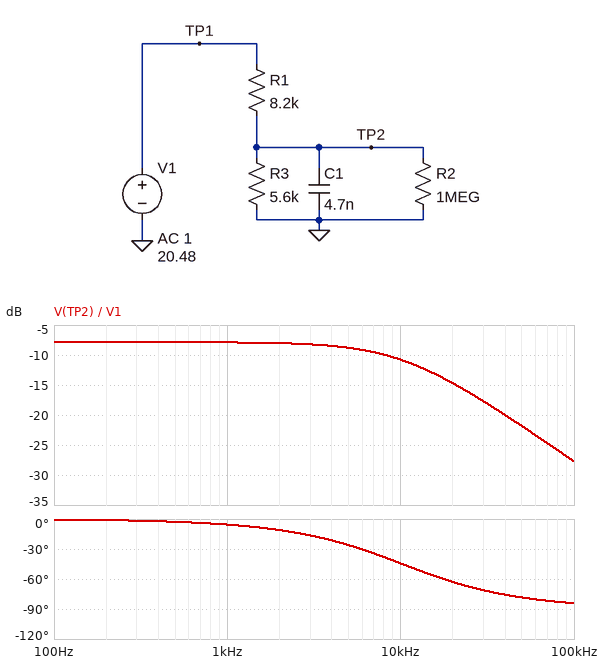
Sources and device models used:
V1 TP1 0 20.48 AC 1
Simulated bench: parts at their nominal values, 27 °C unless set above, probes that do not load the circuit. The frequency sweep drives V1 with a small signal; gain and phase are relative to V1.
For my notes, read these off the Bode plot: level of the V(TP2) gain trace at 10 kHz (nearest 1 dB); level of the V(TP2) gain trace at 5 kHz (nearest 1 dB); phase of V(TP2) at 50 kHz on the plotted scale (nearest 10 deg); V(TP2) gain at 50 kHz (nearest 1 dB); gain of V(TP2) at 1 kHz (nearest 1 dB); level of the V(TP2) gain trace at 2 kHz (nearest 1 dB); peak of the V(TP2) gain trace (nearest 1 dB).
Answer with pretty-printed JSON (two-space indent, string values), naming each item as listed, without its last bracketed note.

{
  "level of the V(TP2) gain trace at 10 kHz": "-11 dB",
  "level of the V(TP2) gain trace at 5 kHz": "-9 dB",
  "phase of V(TP2) at 50 kHz on the plotted scale": "-80 deg",
  "V(TP2) gain at 50 kHz": "-22 dB",
  "gain of V(TP2) at 1 kHz": "-8 dB",
  "level of the V(TP2) gain trace at 2 kHz": "-8 dB",
  "peak of the V(TP2) gain trace": "-8 dB"
}
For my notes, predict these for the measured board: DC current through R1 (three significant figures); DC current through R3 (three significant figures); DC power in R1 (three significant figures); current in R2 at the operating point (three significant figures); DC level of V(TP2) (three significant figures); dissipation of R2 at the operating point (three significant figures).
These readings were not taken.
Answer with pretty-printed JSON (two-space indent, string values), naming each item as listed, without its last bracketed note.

{
  "DC current through R1": "1.49 mA",
  "DC current through R3": "1.48 mA",
  "DC power in R1": "18.1 mW",
  "current in R2 at the operating point": "8.28 µA",
  "DC level of V(TP2)": "8.28 V",
  "dissipation of R2 at the operating point": "68.6 µW"
}
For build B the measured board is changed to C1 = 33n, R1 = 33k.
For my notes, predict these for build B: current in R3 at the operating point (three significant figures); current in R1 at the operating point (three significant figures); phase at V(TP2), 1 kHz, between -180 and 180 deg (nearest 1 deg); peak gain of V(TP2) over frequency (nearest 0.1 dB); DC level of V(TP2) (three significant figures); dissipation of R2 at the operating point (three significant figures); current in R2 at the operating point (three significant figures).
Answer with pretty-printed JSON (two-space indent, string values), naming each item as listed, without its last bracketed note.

{
  "current in R3 at the operating point": "528 µA",
  "current in R1 at the operating point": "531 µA",
  "phase at V(TP2), 1 kHz, between -180 and 180 deg": "-45 deg",
  "peak gain of V(TP2) over frequency": "-16.8 dB",
  "DC level of V(TP2)": "2.96 V",
  "dissipation of R2 at the operating point": "8.74 µW",
  "current in R2 at the operating point": "2.96 µA"
}
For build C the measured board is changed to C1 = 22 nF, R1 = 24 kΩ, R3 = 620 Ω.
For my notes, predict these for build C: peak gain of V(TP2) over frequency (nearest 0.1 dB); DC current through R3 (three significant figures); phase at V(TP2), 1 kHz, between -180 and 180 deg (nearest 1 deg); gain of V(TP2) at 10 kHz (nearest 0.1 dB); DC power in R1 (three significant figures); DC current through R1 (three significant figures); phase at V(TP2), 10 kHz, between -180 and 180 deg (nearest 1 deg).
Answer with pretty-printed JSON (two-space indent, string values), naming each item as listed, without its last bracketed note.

{
  "peak gain of V(TP2) over frequency": "-32.0 dB",
  "DC current through R3": "831 µA",
  "phase at V(TP2), 1 kHz, between -180 and 180 deg": "-5 deg",
  "gain of V(TP2) at 10 kHz": "-34.3 dB",
  "DC power in R1": "16.6 mW",
  "DC current through R1": "832 µA",
  "phase at V(TP2), 10 kHz, between -180 and 180 deg": "-40 deg"
}
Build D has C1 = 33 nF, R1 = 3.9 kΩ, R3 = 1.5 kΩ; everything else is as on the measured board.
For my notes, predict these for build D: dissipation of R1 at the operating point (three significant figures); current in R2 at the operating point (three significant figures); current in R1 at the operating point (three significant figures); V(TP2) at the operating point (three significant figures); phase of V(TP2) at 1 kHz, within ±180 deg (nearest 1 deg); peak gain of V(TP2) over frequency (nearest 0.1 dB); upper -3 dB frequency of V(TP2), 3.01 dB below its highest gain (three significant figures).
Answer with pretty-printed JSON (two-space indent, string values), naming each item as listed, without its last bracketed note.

{
  "dissipation of R1 at the operating point": "56.1 mW",
  "current in R2 at the operating point": "5.68 µA",
  "current in R1 at the operating point": "3.79 mA",
  "V(TP2) at the operating point": "5.68 V",
  "phase of V(TP2) at 1 kHz, within ±180 deg": "-13 deg",
  "peak gain of V(TP2) over frequency": "-11.1 dB",
  "upper -3 dB frequency of V(TP2), 3.01 dB below its highest gain": "4.46 kHz"
}
